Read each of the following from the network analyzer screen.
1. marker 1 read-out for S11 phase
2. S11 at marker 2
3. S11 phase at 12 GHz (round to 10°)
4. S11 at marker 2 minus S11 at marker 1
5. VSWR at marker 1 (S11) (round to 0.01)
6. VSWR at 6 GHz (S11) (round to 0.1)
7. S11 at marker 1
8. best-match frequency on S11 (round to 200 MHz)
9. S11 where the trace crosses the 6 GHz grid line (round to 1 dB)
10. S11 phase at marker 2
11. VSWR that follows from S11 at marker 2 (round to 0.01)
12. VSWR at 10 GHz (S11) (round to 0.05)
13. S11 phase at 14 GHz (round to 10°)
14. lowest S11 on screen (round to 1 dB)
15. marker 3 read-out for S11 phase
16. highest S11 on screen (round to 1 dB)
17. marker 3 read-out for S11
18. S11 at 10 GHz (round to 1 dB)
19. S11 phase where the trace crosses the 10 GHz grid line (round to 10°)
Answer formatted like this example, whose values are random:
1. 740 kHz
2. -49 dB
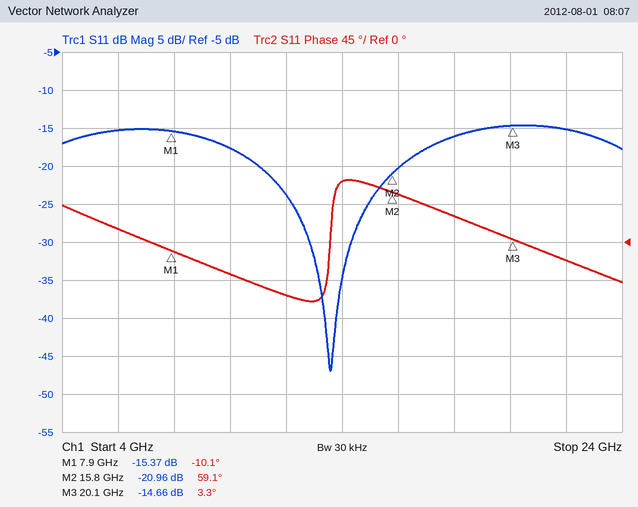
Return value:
1. -10.1°
2. -20.96 dB
3. -60°
4. -5.59 dB
5. 1.41
6. 1.4
7. -15.37 dB
8. 13.6 GHz
9. -15 dB
10. 59.1°
11. 1.20
12. 1.30
13. 70°
14. -47 dB
15. 3.3°
16. -15 dB
17. -14.66 dB
18. -18 dB
19. -40°
